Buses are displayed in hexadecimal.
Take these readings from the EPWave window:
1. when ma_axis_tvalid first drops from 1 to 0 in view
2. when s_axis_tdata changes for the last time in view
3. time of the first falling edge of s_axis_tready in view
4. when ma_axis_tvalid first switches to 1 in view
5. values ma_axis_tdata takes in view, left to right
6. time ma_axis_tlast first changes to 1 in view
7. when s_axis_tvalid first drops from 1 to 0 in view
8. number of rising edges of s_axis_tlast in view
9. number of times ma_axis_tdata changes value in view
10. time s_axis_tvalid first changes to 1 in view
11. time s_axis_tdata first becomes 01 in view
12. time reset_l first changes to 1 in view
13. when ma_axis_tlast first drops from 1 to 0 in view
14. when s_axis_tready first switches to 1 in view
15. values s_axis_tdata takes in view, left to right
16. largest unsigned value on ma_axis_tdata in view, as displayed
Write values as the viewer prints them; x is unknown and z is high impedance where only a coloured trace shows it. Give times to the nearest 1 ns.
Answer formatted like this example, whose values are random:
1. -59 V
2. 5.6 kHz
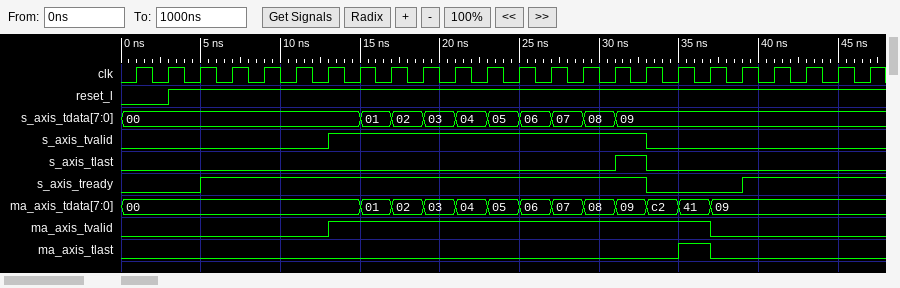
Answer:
1. 37 ns
2. 31 ns
3. 33 ns
4. 13 ns
5. 00, 01, 02, 03, 04, 05, 06, 07, 08, 09, c2, 41, 09
6. 35 ns
7. 33 ns
8. 1
9. 12
10. 13 ns
11. 15 ns
12. 3 ns
13. 37 ns
14. 5 ns
15. 00, 01, 02, 03, 04, 05, 06, 07, 08, 09
16. c2
